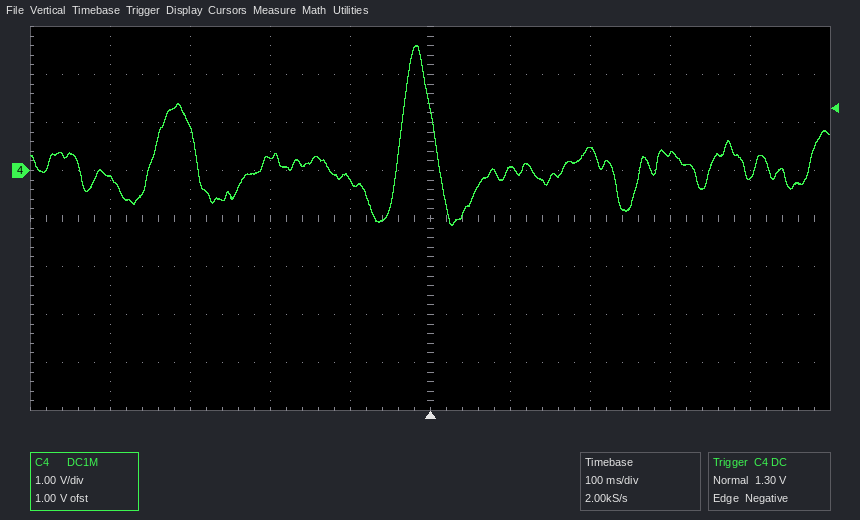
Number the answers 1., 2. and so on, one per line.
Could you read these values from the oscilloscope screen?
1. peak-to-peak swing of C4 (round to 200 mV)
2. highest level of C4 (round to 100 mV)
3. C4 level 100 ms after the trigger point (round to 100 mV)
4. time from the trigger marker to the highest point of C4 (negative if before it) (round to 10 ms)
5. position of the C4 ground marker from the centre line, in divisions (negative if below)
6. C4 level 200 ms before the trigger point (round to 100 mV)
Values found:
1. 3.8 V
2. 2.6 V
3. 0.0 V
4. -20 ms
5. +1.0 div
6. 300 mV
